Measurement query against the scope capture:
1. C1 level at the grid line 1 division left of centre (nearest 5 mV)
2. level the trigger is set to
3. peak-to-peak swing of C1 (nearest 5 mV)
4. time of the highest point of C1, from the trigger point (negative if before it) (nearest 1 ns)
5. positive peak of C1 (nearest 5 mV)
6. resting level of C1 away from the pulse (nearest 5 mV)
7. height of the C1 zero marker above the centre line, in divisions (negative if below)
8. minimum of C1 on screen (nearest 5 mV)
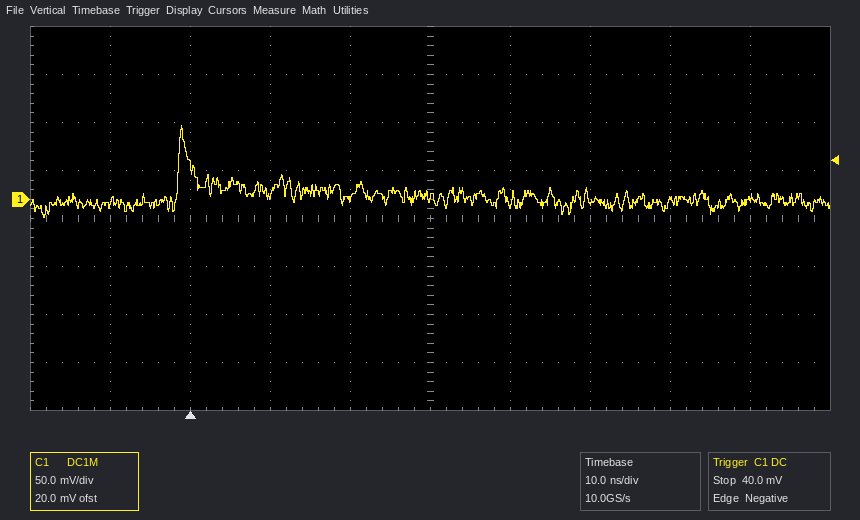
0 mV
40.0 mV
95 mV
-1 ns
75 mV
0 mV
+0.4 div
-20 mV
